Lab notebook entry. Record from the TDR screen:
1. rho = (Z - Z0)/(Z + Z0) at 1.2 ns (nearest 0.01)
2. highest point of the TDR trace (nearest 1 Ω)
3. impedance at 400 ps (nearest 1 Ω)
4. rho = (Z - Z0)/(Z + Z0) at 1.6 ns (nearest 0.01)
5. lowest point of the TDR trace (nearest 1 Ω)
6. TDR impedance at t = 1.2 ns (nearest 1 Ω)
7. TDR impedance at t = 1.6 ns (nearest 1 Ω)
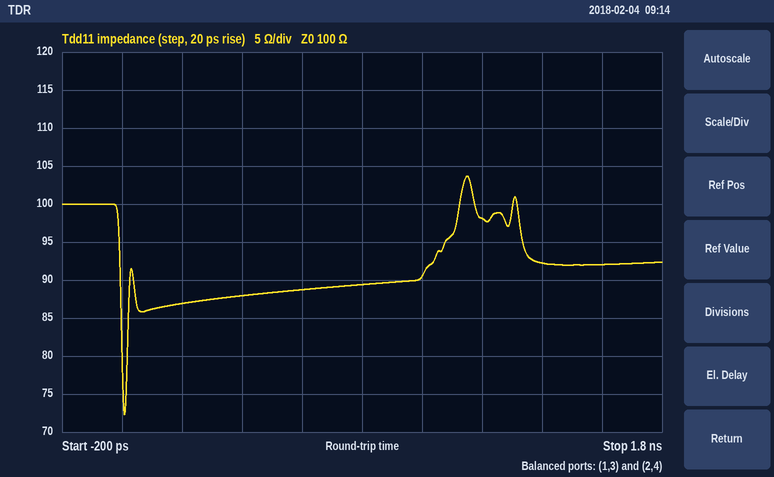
-0.01
104 Ω
88 Ω
-0.04
72 Ω
98 Ω
92 Ω
